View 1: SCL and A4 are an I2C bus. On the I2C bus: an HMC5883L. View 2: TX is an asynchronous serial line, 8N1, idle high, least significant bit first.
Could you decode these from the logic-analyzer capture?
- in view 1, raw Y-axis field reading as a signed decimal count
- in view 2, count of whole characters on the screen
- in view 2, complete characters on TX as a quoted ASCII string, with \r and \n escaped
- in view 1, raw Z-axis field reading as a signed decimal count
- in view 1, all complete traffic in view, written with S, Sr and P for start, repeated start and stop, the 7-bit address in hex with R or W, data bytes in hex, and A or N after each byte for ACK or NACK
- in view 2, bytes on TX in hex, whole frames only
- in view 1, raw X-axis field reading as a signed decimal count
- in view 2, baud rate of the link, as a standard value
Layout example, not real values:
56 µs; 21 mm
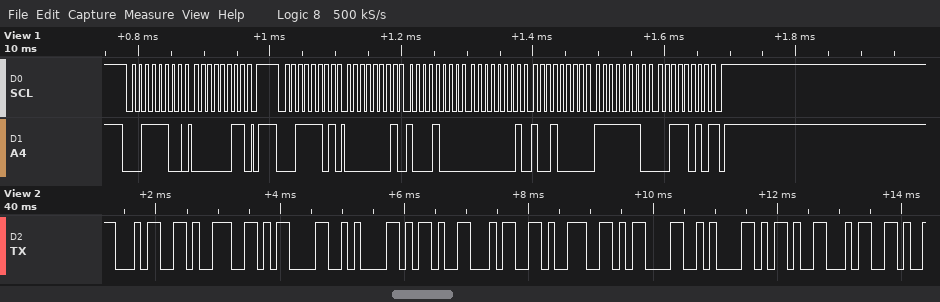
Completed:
-454; 11; "49\r\n-49\r\n-4"; 400; S 1EW A 03 A P S 1ER A 01 A 88 A 01 A 90 A FE A 3A N P; 34 39 0D 0A 2D 34 39 0D 0A 2D 34; 392; 9600 baud
